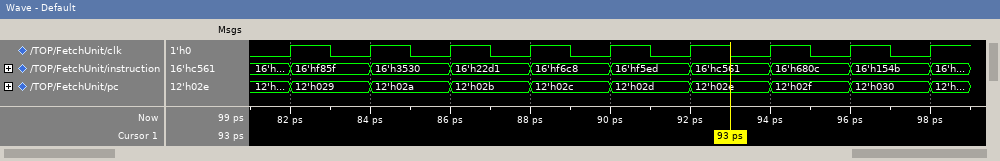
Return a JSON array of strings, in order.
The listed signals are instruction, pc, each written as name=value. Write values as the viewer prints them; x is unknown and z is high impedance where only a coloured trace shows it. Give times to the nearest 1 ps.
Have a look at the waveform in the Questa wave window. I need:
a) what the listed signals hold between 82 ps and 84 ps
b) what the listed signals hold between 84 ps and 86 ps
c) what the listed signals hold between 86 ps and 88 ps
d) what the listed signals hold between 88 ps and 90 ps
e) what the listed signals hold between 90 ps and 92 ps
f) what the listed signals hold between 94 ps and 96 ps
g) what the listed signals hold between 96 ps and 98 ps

["instruction=16'hf85f, pc=12'h029", "instruction=16'h3530, pc=12'h02a", "instruction=16'h22d1, pc=12'h02b", "instruction=16'hf6c8, pc=12'h02c", "instruction=16'hf5ed, pc=12'h02d", "instruction=16'h680c, pc=12'h02f", "instruction=16'h154b, pc=12'h030"]
